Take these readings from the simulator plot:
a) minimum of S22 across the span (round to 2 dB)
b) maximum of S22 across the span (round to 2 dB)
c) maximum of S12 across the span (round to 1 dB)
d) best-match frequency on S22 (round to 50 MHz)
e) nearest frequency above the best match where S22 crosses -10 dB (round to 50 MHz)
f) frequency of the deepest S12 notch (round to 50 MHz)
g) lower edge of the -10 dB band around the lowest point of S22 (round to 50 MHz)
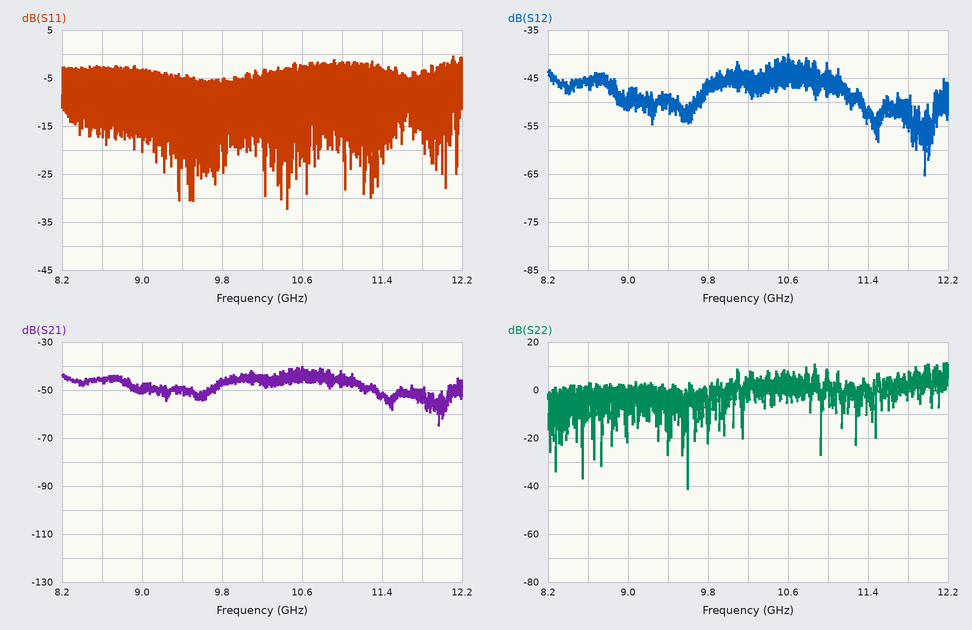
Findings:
-42 dB
12 dB
-40 dB
9.60 GHz
9.60 GHz
11.95 GHz
9.60 GHz
